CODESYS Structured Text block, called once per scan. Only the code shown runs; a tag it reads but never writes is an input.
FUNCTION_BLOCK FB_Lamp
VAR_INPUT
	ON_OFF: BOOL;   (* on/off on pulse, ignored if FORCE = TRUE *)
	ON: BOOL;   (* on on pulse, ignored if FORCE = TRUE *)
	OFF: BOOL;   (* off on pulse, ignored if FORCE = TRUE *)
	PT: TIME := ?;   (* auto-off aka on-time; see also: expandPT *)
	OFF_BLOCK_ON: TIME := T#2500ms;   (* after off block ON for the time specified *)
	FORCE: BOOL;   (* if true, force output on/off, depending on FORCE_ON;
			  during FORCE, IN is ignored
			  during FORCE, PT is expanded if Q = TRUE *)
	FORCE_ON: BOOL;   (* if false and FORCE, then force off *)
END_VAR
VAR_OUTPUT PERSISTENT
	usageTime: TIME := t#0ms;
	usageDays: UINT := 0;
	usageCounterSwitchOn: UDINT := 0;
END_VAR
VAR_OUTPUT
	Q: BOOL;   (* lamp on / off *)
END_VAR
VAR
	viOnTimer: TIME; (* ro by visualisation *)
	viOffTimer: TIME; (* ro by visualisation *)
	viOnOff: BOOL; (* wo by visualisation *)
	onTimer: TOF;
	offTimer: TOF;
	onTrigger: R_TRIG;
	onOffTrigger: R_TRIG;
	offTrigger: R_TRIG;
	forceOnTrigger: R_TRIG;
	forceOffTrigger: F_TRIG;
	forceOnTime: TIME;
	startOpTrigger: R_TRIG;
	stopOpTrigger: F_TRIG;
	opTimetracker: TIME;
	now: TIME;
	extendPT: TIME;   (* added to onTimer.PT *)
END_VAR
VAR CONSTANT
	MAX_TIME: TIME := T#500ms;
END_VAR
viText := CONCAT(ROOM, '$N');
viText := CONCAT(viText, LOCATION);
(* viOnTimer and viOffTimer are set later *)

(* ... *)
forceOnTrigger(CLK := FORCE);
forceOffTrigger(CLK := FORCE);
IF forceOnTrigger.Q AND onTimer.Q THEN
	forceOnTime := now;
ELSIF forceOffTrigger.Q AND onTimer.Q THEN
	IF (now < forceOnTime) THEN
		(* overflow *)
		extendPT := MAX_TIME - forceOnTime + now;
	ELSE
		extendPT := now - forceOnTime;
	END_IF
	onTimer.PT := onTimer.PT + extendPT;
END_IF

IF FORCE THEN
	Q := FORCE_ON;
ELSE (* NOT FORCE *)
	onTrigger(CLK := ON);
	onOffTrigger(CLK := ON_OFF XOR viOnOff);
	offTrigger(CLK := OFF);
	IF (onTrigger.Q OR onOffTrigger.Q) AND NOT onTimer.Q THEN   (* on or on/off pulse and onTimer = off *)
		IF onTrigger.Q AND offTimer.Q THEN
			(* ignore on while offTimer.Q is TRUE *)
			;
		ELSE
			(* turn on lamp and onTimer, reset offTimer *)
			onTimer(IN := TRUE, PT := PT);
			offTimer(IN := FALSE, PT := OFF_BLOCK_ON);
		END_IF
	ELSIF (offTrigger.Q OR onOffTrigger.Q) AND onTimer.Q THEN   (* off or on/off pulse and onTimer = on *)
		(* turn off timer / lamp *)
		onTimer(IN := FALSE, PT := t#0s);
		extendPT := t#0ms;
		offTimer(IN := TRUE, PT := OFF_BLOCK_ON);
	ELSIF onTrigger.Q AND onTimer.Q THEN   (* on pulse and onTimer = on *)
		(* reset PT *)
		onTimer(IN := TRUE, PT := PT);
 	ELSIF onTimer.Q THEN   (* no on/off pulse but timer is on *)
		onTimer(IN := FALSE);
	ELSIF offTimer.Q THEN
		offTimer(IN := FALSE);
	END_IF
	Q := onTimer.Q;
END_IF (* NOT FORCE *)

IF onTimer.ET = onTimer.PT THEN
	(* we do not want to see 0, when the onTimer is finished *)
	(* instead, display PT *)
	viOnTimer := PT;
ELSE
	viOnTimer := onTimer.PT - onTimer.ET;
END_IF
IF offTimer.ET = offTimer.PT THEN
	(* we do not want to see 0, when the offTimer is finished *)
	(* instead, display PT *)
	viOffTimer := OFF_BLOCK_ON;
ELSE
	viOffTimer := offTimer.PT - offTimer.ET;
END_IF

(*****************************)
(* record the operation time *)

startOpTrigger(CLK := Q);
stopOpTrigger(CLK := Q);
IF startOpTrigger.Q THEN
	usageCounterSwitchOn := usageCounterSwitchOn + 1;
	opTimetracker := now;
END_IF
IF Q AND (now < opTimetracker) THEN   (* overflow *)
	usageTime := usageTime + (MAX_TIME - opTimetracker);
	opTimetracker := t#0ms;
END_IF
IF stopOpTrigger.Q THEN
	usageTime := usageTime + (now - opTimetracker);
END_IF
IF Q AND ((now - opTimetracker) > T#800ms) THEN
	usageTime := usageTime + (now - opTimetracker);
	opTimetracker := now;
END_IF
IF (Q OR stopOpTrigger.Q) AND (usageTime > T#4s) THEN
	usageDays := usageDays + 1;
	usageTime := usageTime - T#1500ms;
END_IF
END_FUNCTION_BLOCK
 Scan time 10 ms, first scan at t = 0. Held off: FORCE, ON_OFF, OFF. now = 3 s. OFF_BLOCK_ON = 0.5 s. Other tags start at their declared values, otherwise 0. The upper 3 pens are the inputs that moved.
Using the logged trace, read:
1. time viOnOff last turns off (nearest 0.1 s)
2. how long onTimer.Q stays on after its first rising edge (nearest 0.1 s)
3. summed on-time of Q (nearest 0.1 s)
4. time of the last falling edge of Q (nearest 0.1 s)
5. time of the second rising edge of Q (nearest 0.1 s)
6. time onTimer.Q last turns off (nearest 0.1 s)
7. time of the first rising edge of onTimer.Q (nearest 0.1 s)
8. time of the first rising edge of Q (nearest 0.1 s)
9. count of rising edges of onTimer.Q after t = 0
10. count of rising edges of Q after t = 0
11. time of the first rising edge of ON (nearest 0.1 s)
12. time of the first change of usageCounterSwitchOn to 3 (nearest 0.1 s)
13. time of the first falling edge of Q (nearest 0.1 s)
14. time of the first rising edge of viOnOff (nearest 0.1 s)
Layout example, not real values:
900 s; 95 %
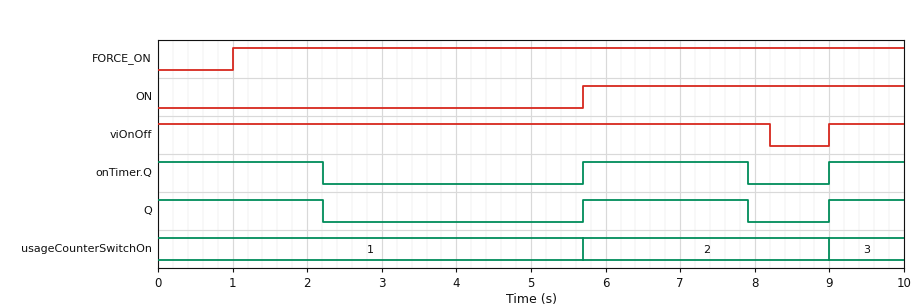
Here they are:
8.2 s; 2.2 s; 5.4 s; 7.9 s; 9.0 s; 7.9 s; 5.7 s; 5.7 s; 2; 2; 5.7 s; 9.0 s; 2.2 s; 9.0 s
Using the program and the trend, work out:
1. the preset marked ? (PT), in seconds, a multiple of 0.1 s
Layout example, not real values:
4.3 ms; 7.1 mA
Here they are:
2.2 s
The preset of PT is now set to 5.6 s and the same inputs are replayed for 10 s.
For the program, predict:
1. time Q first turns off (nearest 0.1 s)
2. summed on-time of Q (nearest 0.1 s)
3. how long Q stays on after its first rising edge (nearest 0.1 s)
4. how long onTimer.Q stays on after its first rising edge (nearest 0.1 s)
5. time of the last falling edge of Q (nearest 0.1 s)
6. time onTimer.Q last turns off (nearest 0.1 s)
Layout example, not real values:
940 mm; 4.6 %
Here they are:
5.6 s; 8.9 s; 3.3 s; 3.3 s; 9.0 s; 9.0 s
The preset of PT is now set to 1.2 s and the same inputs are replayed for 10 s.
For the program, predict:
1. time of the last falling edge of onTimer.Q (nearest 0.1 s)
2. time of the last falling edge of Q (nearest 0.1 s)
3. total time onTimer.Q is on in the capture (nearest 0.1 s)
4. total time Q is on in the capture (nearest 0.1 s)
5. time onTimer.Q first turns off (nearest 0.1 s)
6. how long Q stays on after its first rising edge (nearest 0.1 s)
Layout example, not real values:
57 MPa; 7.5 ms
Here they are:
6.9 s; 6.9 s; 3.4 s; 3.4 s; 1.2 s; 1.2 s
